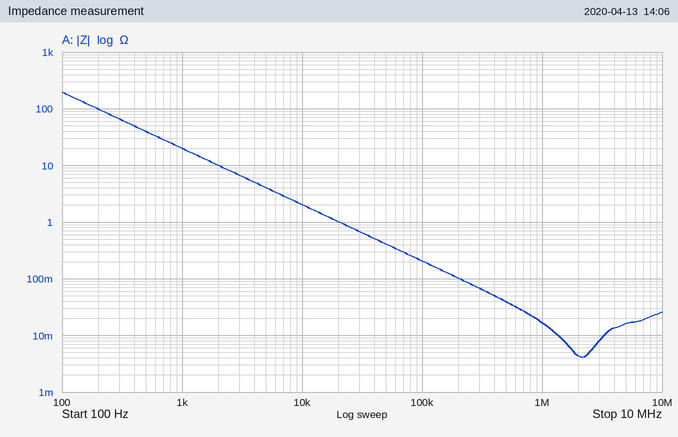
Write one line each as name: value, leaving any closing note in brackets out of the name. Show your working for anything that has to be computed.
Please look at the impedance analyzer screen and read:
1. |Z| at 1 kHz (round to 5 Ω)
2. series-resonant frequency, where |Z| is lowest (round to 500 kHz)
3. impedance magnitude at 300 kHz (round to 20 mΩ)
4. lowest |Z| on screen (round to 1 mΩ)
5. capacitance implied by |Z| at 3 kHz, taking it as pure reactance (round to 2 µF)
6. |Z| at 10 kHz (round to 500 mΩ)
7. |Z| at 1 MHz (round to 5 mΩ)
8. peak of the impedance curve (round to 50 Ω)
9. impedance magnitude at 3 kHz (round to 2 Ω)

|Z| at 1 kHz: 20 Ω
series-resonant frequency, where |Z| is lowest: 2.0 MHz
impedance magnitude at 300 kHz: 60 mΩ
lowest |Z| on screen: 4 mΩ
capacitance implied by |Z| at 3 kHz, taking it as pure reactance: C = 1/(2π × 3 kHz × 6 Ω) ≈ 8.84 µF, so 8 µF to the nearest 2 µF
|Z| at 10 kHz: 2.0 Ω
|Z| at 1 MHz: 15 mΩ
peak of the impedance curve: 200 Ω
impedance magnitude at 3 kHz: 6 Ω
